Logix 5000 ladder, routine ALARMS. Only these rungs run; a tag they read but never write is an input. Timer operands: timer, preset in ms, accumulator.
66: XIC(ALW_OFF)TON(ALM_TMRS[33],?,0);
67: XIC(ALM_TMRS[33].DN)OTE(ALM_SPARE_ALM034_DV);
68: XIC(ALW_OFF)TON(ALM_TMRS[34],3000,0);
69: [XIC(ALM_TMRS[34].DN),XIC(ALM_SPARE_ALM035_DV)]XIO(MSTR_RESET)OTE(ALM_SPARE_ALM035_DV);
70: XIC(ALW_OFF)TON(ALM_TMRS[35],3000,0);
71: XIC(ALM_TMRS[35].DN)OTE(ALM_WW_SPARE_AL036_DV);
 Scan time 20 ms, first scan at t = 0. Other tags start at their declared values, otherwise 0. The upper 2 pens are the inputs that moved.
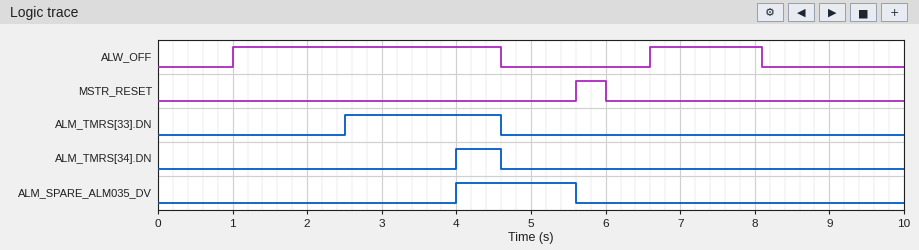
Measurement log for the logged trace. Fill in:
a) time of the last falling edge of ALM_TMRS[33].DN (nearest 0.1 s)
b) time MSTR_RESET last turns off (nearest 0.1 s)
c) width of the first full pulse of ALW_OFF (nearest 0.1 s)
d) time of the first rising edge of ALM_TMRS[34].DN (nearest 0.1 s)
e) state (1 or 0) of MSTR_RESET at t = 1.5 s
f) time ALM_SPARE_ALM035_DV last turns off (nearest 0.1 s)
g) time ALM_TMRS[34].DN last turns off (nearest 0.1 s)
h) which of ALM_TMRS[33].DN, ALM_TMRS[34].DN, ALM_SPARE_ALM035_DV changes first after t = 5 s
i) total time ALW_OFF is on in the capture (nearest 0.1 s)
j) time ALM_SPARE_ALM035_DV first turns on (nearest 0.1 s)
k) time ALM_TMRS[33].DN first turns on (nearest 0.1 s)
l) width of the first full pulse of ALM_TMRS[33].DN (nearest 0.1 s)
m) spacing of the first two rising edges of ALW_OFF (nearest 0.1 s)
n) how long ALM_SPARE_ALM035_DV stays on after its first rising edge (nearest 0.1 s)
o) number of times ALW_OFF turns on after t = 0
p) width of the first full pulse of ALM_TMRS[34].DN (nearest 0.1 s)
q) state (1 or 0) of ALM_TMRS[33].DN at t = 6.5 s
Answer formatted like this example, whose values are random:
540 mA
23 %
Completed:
4.6 s
6.0 s
3.6 s
4.0 s
0
5.6 s
4.6 s
ALM_SPARE_ALM035_DV
5.1 s
4.0 s
2.5 s
2.1 s
5.6 s
1.6 s
2
0.6 s
0
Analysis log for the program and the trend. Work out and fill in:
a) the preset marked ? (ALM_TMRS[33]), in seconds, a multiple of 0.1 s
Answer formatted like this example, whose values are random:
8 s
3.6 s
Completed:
1.5 s
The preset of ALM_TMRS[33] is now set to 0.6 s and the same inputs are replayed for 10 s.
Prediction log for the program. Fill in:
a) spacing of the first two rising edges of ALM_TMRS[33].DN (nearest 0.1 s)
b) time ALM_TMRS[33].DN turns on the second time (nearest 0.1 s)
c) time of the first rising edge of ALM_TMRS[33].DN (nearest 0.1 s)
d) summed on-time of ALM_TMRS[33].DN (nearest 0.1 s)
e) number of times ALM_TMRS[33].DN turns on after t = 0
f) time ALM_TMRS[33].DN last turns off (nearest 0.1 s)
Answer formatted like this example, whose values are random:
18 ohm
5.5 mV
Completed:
5.6 s
7.2 s
1.6 s
3.9 s
2
8.1 s
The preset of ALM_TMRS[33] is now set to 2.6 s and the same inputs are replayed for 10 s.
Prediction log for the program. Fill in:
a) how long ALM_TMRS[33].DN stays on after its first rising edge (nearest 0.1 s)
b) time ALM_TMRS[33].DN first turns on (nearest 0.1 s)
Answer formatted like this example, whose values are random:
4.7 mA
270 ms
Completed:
1.0 s
3.6 s
